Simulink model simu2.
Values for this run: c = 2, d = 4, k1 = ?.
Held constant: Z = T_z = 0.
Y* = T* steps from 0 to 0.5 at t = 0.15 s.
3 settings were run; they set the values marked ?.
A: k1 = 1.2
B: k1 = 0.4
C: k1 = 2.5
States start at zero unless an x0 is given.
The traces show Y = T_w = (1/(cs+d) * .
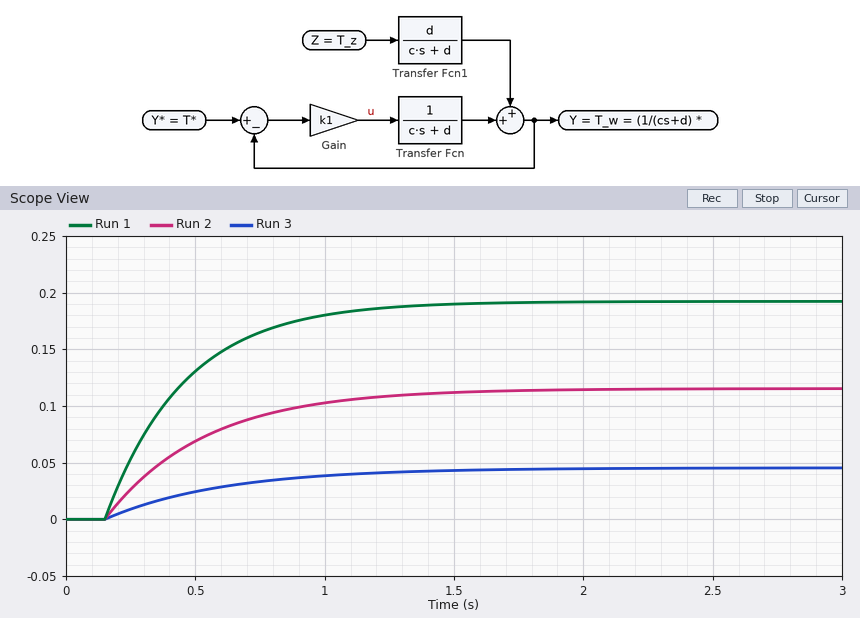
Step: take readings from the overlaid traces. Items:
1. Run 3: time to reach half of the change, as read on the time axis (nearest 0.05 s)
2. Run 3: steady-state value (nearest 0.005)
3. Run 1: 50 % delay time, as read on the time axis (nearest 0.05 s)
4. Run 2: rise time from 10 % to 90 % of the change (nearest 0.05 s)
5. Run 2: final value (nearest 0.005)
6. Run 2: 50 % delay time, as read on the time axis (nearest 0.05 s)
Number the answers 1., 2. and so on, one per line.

1. 0.45 s
2. 0.045
3. 0.35 s
4. 0.85 s
5. 0.115
6. 0.40 s
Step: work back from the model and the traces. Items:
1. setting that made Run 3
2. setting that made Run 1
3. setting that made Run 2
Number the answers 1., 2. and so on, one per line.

1. B
2. C
3. A
